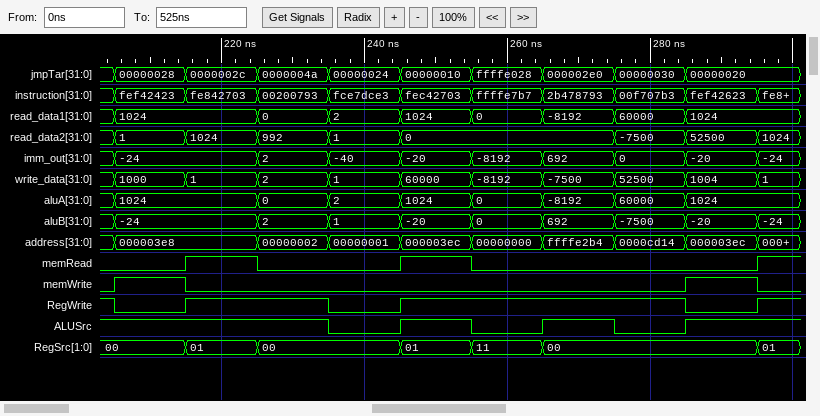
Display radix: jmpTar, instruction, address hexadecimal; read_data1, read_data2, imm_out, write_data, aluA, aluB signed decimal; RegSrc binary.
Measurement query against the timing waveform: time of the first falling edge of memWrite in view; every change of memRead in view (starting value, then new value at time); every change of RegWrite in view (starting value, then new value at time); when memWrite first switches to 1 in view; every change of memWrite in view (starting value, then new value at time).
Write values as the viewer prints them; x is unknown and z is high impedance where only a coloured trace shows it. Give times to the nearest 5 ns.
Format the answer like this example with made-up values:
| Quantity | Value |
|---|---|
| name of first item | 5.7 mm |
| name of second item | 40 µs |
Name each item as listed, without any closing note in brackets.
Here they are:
| Quantity | Value |
|---|---|
| time of the first falling edge of memWrite in view | 215 ns |
| every change of memRead in view | 0, 1 at 215 ns, 0 at 225 ns, 1 at 245 ns, 0 at 255 ns, 1 at 295 ns |
| every change of RegWrite in view | 1, 0 at 205 ns, 1 at 215 ns, 0 at 235 ns, 1 at 245 ns, 0 at 285 ns, 1 at 295 ns |
| when memWrite first switches to 1 in view | 205 ns |
| every change of memWrite in view | 0, 1 at 205 ns, 0 at 215 ns, 1 at 285 ns, 0 at 295 ns |
